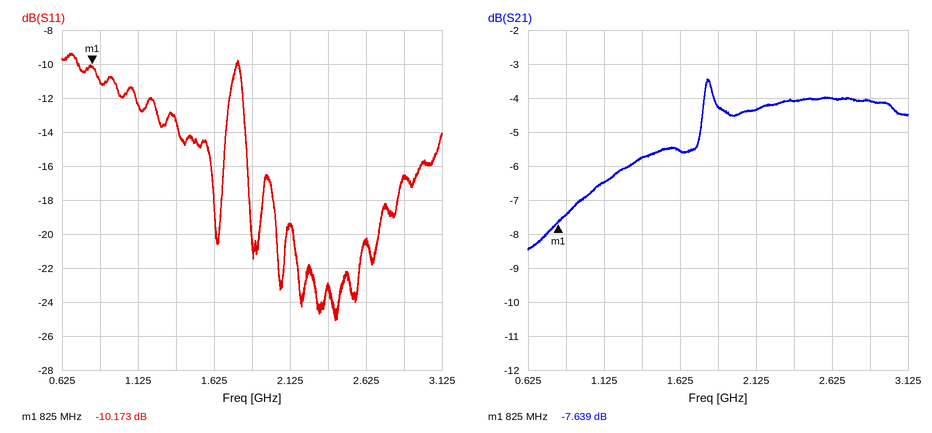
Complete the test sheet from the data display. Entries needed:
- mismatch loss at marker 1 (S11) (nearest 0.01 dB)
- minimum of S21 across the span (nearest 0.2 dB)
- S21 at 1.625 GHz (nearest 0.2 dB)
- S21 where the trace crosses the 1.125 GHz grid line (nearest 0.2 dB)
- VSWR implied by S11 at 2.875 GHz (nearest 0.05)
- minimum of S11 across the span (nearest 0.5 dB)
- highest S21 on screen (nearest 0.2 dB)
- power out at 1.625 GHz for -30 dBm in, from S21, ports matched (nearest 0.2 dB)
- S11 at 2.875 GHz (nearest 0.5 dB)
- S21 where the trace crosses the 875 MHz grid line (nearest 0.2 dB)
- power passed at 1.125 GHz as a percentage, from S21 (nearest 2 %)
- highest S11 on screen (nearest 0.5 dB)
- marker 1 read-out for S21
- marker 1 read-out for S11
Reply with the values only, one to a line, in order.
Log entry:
0.44 dB
-8.4 dB
-5.6 dB
-6.4 dB
1.35
-25.0 dB
-3.4 dB
-35.6 dBm
-16.5 dB
-7.4 dB
22 %
-9.5 dB
-7.639 dB
-10.173 dB
